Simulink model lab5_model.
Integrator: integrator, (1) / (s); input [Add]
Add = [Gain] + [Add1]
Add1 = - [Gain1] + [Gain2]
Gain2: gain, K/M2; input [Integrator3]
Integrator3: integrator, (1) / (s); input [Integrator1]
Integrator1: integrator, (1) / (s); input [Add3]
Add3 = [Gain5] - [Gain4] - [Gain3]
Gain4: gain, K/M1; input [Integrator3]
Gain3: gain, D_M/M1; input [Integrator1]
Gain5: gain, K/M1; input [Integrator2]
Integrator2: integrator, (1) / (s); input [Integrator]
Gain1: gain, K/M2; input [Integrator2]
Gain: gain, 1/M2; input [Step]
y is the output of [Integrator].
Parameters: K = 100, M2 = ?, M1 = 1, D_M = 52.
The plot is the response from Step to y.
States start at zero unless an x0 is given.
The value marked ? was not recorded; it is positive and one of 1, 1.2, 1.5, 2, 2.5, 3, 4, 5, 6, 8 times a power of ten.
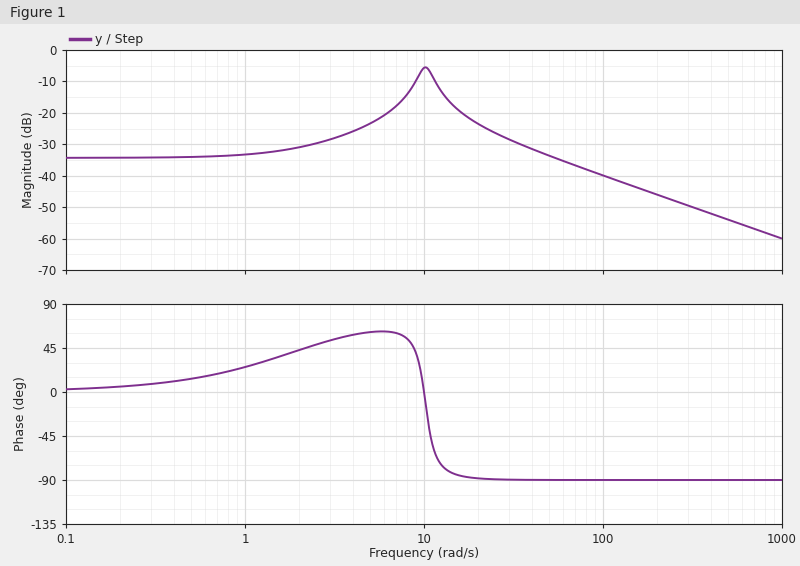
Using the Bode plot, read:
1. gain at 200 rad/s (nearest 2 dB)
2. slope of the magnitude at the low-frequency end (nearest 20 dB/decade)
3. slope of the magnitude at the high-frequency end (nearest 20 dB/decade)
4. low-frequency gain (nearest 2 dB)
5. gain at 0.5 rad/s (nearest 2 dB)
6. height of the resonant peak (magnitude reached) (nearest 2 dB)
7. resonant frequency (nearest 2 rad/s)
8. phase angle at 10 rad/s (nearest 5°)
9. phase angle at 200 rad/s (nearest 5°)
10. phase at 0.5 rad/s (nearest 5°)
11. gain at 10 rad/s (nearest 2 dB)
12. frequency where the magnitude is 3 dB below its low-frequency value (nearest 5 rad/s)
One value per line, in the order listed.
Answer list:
-46 dB
0 dB/decade
-20 dB/decade
-34 dB
-34 dB
-6 dB
10 rad/s
0°
-90°
15°
-6 dB
75 rad/s
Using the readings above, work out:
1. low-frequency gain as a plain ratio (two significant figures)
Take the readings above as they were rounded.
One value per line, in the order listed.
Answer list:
0.020
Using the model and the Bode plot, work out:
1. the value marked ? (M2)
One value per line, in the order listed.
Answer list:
1
